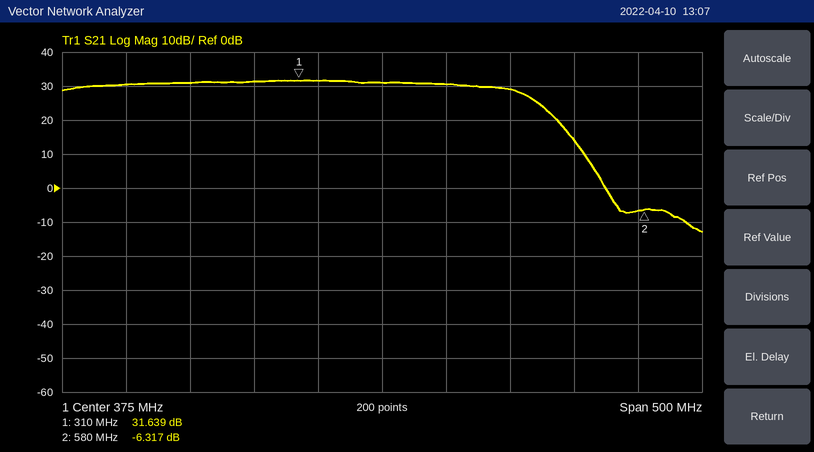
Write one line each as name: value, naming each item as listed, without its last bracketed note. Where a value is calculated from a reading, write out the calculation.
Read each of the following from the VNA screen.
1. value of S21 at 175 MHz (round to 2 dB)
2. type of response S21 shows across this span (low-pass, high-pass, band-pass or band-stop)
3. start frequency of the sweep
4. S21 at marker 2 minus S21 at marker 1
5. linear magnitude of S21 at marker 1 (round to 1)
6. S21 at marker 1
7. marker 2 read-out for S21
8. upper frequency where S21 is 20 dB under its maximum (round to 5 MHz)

value of S21 at 175 MHz: 30 dB
type of response S21 shows across this span: low-pass
start frequency of the sweep: 125 MHz
S21 at marker 2 minus S21 at marker 1: -6.317 − (31.639) = -37.956 dB
linear magnitude of S21 at marker 1: 10^(31.639/20) ≈ 38
S21 at marker 1: 31.639 dB
marker 2 read-out for S21: -6.317 dB
upper frequency where S21 is 20 dB under its maximum: 530 MHz
